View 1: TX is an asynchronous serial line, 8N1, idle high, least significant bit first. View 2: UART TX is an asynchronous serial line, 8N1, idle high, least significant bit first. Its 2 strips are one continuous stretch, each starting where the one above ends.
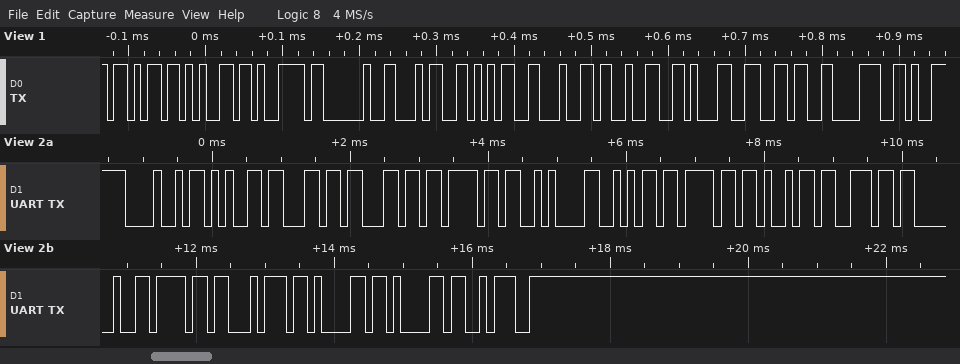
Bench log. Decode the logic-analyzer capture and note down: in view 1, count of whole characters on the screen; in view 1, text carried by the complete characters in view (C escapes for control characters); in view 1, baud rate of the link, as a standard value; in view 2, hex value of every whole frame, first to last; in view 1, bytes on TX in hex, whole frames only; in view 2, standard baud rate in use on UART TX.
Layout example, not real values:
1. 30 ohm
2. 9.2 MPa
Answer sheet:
1. 11
2. "key 45d2168"
3. 115200 baud
4. 48 65 6C 6C 6F 0A 6A 6F 69 6E 20 6F 74 61 61 3A
5. 6B 65 79 20 34 35 64 32 31 36 38
6. 9600 baud
